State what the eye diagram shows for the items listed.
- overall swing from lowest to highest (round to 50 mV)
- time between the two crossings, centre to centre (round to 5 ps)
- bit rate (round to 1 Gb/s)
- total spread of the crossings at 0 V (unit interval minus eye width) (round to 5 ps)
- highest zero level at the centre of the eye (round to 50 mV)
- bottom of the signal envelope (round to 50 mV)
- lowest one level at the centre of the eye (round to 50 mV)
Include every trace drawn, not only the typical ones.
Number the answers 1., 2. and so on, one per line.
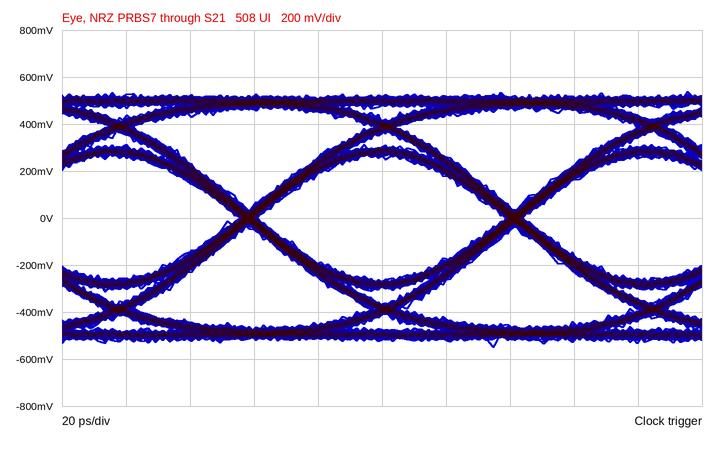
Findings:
1. 1.10 V
2. 85 ps
3. 12 Gb/s
4. 5 ps
5. -250 mV
6. -550 mV
7. 250 mV
